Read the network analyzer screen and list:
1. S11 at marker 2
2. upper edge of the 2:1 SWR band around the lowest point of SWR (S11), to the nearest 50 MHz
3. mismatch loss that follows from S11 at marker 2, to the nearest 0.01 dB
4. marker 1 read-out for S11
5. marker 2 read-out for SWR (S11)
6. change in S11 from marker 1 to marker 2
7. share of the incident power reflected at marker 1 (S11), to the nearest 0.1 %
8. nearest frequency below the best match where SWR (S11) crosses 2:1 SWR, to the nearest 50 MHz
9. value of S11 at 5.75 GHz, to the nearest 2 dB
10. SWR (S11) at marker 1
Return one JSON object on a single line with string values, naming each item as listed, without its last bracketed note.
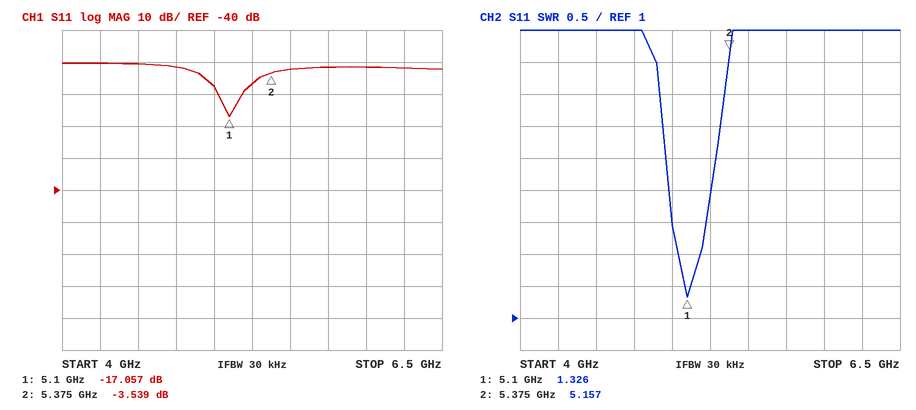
{"S11 at marker 2": "-3.539 dB", "upper edge of the 2:1 SWR band around the lowest point of SWR (S11), to the nearest 50 MHz": "5.20 GHz", "mismatch loss that follows from S11 at marker 2, to the nearest 0.01 dB": "2.54 dB", "marker 1 read-out for S11": "-17.057 dB", "marker 2 read-out for SWR": "5.157", "change in S11 from marker 1 to marker 2": "13.518 dB", "share of the incident power reflected at marker 1 (S11), to the nearest 0.1 %": "2.0 %", "nearest frequency below the best match where SWR (S11) crosses 2:1 SWR, to the nearest 50 MHz": "5.05 GHz", "value of S11 at 5.75 GHz, to the nearest 2 dB": "-2 dB", "SWR (S11) at marker 1": "1.326"}
